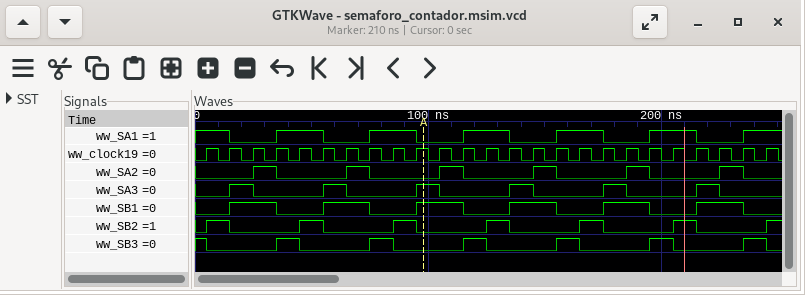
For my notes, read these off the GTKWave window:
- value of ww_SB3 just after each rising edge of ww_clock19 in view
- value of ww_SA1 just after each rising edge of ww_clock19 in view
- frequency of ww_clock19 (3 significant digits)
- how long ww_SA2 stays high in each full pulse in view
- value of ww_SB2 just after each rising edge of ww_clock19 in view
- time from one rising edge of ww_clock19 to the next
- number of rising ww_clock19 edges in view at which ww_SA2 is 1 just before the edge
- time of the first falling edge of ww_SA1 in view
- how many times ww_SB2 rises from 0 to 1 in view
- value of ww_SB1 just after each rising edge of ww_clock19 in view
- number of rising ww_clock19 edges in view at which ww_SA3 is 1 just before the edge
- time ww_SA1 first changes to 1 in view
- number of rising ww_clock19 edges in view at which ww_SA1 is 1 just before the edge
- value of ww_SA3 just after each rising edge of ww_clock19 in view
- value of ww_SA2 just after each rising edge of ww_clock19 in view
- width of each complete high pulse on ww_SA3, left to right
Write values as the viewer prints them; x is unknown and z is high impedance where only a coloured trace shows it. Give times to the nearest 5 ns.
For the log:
0 0 0 1 0 0 0 1 0 0 0 1 0 0 0 1 0 0 0 1 0 0 0 1 0
1 0 0 1 1 0 0 1 1 0 0 1 1 0 0 1 1 0 0 1 1 0 0 1 1
100 MHz
10 ns, 10 ns, 10 ns, 10 ns, 10 ns, 10 ns
1 0 0 0 1 0 0 0 1 0 0 0 1 0 0 0 1 0 0 0 1 0 0 0 1
10 ns
6
15 ns
7
0 1 1 0 0 1 1 0 0 1 1 0 0 1 1 0 0 1 1 0 0 1 1 0 0
6
35 ns
13
0 1 0 0 0 1 0 0 0 1 0 0 0 1 0 0 0 1 0 0 0 1 0 0 0
0 0 1 0 0 0 1 0 0 0 1 0 0 0 1 0 0 0 1 0 0 0 1 0 0
10 ns, 10 ns, 10 ns, 10 ns, 10 ns, 10 ns
